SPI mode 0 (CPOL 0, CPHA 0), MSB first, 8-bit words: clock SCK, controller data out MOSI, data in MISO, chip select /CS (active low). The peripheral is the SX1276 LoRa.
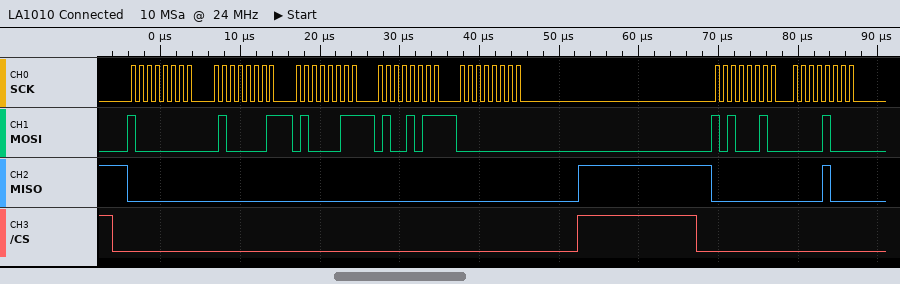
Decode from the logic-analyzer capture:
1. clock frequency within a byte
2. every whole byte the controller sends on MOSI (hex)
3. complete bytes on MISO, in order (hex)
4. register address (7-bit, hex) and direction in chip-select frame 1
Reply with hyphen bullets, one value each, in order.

- 1 MHz
- 0x80 0x41 0x43 0x4B 0x00 0xA2 0x08
- 0x00 0x00 0x00 0x00 0x00 0x00 0x08
- 0x00 write
